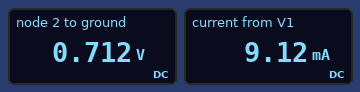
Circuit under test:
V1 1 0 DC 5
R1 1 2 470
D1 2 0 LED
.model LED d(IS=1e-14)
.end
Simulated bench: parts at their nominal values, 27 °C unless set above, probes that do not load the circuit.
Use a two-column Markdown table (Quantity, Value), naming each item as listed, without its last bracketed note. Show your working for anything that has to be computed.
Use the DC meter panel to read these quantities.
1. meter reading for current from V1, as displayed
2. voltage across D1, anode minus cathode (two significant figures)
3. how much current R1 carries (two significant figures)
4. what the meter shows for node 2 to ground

| Quantity | Value |
|---|---|
| meter reading for current from V1, as displayed | 9.12 mA |
| voltage across D1, anode minus cathode | 712 mV = 710 mV |
| how much current R1 carries | (5 V - 712 mV) / 470 Ω = 9.1 mA |
| what the meter shows for node 2 to ground | 0.712 V |
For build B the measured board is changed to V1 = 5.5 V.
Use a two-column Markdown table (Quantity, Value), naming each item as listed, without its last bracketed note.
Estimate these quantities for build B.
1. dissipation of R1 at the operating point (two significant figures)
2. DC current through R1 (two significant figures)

| Quantity | Value |
|---|---|
| dissipation of R1 at the operating point | 49 mW |
| DC current through R1 | 10 mA |
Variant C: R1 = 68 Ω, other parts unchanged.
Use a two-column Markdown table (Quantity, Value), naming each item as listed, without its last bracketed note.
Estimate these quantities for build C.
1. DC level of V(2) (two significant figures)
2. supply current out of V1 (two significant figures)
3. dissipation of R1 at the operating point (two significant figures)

| Quantity | Value |
|---|---|
| DC level of V(2) | 760 mV |
| supply current out of V1 | 62 mA |
| dissipation of R1 at the operating point | 260 mW |
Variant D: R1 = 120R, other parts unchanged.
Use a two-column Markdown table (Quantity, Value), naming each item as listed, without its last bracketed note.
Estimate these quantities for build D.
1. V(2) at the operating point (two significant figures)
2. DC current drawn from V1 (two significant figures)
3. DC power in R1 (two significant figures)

| Quantity | Value |
|---|---|
| V(2) at the operating point | 750 mV |
| DC current drawn from V1 | 35 mA |
| DC power in R1 | 150 mW |
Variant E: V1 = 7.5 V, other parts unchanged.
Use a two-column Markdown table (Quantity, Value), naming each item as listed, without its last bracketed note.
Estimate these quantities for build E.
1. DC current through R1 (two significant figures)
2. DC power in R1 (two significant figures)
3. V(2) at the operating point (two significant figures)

| Quantity | Value |
|---|---|
| DC current through R1 | 14 mA |
| DC power in R1 | 98 mW |
| V(2) at the operating point | 720 mV |
